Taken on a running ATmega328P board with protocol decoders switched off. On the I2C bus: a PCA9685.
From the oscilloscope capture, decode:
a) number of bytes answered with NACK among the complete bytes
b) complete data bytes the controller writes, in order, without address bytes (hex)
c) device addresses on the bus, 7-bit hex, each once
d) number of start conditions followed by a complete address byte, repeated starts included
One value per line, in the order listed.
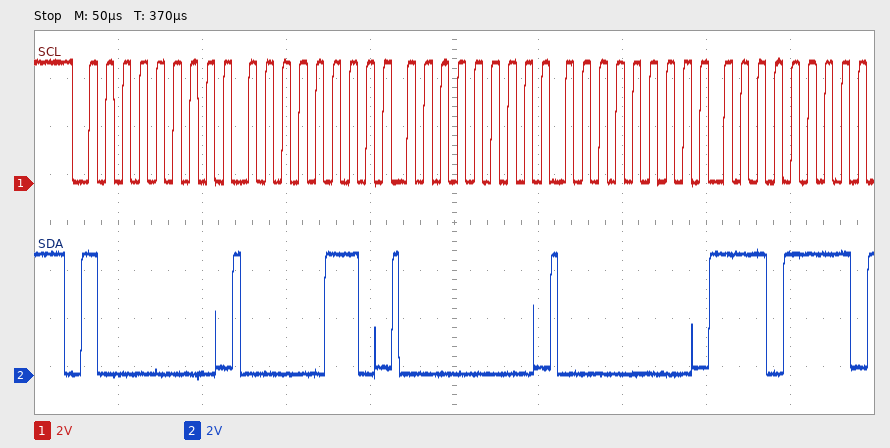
0
06 00 00 EF
0x40
1
